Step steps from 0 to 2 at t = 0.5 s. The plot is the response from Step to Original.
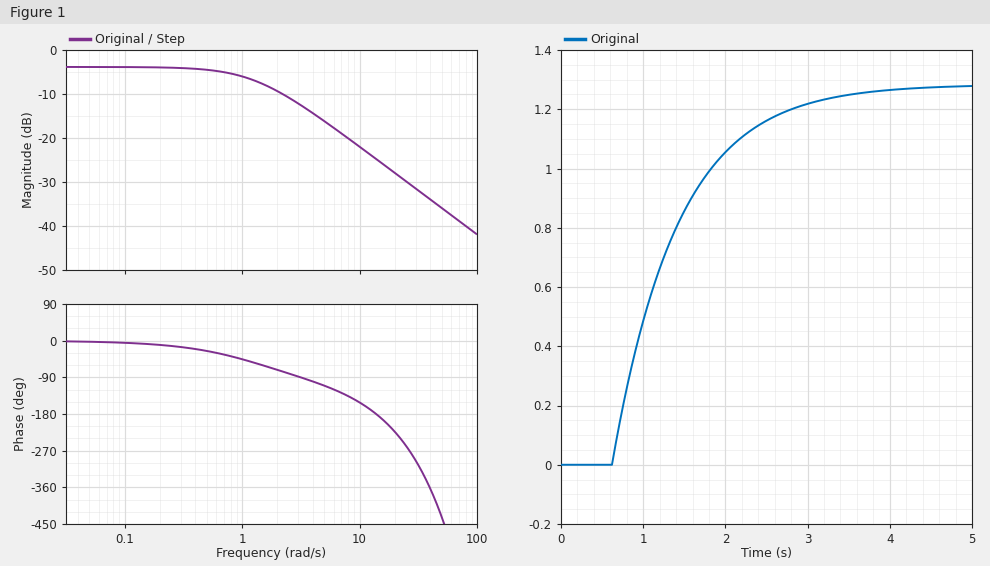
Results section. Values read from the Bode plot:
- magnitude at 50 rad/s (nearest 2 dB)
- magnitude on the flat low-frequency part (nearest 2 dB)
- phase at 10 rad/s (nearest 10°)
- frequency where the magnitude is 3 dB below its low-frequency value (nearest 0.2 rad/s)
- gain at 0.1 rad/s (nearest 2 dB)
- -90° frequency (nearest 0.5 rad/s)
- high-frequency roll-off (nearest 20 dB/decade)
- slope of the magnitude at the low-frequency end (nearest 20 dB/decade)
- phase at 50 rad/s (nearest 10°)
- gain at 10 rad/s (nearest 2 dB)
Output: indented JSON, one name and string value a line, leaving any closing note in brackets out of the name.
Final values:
{
  "magnitude at 50 rad/s": "-36 dB",
  "magnitude on the flat low-frequency part": "-4 dB",
  "phase at 10 rad/s": "-150°",
  "frequency where the magnitude is 3 dB below its low-frequency value": "1.2 rad/s",
  "gain at 0.1 rad/s": "-4 dB",
  "-90° frequency": "3.0 rad/s",
  "high-frequency roll-off": "-20 dB/decade",
  "slope of the magnitude at the low-frequency end": "0 dB/decade",
  "phase at 50 rad/s": "-430°",
  "gain at 10 rad/s": "-22 dB"
}
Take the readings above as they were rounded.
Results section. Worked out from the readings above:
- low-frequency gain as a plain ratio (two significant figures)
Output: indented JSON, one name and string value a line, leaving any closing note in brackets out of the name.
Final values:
{
  "low-frequency gain as a plain ratio": "0.63"
}
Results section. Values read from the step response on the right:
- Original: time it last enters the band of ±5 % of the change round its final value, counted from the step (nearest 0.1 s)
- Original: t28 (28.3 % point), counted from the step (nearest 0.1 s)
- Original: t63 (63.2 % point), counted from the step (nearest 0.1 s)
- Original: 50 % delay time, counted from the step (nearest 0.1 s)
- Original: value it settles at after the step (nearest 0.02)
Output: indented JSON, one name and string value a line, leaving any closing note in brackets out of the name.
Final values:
{
  "Original: time it last enters the band of ±5 % of the change round its final value, counted from the step": "2.5 s",
  "Original: t28 (28.3 % point), counted from the step": "0.4 s",
  "Original: t63 (63.2 % point), counted from the step": "0.9 s",
  "Original: 50 % delay time, counted from the step": "0.7 s",
  "Original: value it settles at after the step": "1.28"
}
